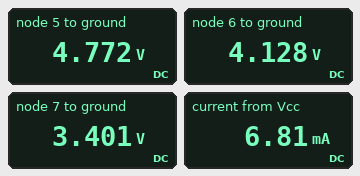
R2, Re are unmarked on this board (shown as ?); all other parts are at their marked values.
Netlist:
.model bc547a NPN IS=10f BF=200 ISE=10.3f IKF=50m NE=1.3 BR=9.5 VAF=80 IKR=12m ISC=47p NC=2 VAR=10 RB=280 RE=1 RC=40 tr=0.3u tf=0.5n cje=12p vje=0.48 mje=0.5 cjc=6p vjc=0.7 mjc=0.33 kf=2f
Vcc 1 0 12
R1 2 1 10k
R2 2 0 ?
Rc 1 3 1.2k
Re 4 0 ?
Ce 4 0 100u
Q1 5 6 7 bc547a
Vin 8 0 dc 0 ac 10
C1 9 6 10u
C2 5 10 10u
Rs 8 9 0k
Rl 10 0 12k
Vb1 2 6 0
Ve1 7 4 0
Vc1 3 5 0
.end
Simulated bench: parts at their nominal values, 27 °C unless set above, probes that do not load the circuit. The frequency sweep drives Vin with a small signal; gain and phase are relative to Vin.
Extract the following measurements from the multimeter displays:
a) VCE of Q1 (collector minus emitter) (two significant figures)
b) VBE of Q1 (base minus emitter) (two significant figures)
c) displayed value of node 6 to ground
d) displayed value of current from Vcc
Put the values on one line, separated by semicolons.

1.4 V; 730 mV; 4.128 V; 6.81 mA
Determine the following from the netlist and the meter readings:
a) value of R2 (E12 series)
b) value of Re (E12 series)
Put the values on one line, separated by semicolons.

5.6 kΩ; 560 Ω
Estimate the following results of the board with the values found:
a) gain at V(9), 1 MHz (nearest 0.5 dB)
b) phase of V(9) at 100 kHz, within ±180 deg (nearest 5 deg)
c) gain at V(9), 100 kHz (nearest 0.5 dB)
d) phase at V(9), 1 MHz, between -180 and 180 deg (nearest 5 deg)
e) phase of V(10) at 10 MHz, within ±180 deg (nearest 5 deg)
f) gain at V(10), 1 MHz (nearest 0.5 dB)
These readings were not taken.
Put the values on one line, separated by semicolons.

0 dB; 0 deg; 0 dB; 0 deg; 90 deg; 37.5 dB
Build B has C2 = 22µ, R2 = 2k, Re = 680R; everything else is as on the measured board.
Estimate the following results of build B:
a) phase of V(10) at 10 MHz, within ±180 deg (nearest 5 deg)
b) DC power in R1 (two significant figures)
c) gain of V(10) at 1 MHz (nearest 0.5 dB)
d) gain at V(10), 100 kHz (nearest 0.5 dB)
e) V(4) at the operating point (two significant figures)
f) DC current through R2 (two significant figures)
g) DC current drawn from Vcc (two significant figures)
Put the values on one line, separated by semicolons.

100 deg; 10 mW; 35.0 dB; 36.0 dB; 1.3 V; 990 µA; 2.9 mA
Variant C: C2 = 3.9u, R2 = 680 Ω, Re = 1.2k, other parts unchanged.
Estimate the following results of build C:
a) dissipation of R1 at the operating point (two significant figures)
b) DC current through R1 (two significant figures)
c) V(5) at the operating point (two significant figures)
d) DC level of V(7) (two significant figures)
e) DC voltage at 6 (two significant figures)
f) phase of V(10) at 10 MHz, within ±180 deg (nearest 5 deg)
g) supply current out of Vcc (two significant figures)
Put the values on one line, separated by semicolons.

13 mW; 1.1 mA; 12 V; 160 mV; 760 mV; 130 deg; 1.3 mA
